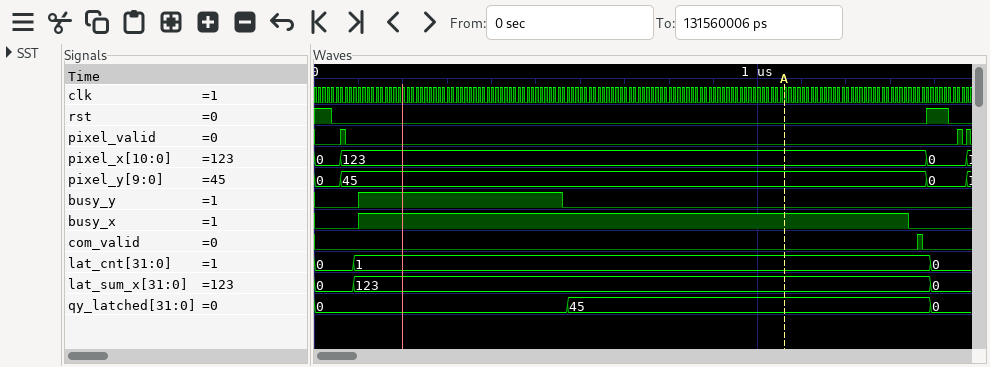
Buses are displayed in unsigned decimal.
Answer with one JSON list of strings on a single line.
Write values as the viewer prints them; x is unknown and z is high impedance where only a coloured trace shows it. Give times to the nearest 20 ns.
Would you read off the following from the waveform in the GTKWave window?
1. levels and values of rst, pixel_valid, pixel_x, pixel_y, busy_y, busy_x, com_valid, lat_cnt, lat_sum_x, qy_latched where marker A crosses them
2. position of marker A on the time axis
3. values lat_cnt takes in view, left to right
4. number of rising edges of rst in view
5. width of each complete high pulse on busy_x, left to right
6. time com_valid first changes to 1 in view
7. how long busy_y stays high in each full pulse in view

["rst=0, pixel_valid=0, pixel_x=123, pixel_y=45, busy_y=0, busy_x=1, com_valid=0, lat_cnt=1, lat_sum_x=123, qy_latched=45", "1060 ns", "0, 1, 0", "1", "1240 ns", "1360 ns", "460 ns"]
